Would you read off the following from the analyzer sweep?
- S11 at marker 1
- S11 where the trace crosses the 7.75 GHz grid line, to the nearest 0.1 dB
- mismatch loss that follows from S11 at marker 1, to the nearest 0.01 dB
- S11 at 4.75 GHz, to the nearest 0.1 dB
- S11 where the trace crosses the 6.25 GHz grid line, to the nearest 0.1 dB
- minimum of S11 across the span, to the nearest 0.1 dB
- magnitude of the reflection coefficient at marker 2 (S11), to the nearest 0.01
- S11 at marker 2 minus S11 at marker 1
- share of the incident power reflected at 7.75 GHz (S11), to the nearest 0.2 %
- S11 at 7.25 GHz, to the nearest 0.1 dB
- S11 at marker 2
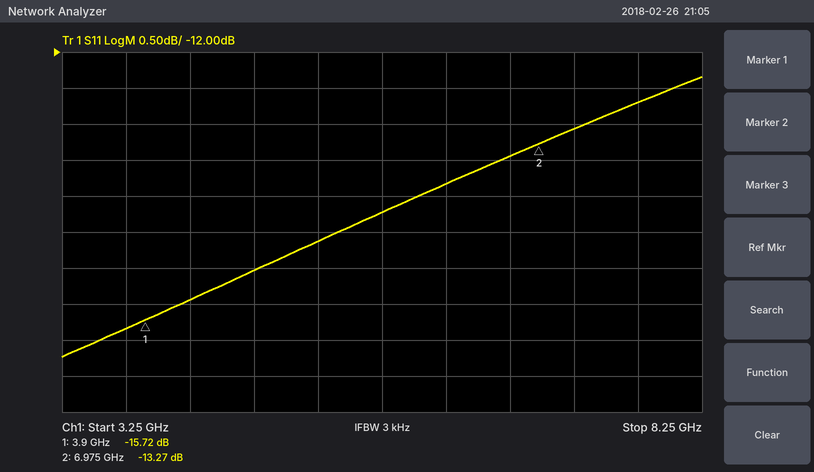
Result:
-15.72 dB
-12.7 dB
0.12 dB
-15.0 dB
-13.8 dB
-16.2 dB
0.22
2.45 dB
5.4 %
-13.1 dB
-13.27 dB
